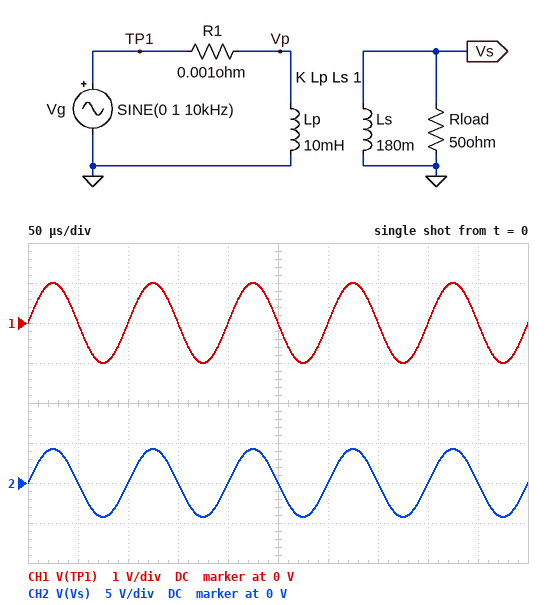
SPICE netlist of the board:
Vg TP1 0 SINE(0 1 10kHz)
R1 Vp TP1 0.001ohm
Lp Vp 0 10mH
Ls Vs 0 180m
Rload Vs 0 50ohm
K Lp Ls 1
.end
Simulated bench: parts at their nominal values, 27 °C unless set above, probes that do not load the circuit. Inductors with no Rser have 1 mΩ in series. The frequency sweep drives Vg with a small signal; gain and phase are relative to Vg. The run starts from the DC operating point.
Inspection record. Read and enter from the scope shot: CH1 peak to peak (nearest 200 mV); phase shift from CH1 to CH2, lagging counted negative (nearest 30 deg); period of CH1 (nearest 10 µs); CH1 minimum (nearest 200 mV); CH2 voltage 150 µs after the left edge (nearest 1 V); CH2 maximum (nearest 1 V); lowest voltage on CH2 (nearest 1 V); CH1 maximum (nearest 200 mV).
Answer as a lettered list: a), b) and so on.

a) 2.0 V
b) 0 deg
c) 100 µs
d) -1.0 V
e) 0 V
f) 4 V
g) -4 V
h) 1.0 V
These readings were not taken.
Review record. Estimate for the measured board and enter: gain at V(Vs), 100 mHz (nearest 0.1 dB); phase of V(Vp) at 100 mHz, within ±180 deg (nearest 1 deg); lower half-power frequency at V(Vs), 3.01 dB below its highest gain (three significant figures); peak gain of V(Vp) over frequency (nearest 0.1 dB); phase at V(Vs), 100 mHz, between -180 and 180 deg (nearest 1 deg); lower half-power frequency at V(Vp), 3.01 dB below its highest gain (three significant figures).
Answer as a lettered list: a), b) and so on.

a) 12.1 dB
b) 9 deg
c) 31.8 mHz
d) 0 dB
e) 18 deg
f) 22.5 mHz
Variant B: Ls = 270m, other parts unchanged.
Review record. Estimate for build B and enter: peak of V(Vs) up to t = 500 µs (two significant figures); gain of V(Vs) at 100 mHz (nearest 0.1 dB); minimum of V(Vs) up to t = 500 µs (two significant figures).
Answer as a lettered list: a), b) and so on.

a) 5.2 V
b) 13.9 dB
c) -5.2 V
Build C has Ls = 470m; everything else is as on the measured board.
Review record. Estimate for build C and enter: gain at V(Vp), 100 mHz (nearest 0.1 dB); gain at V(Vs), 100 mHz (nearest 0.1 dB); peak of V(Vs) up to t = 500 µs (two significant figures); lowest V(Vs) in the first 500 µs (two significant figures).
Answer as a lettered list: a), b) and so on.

a) -0.3 dB
b) 16.3 dB
c) 6.8 V
d) -6.8 V
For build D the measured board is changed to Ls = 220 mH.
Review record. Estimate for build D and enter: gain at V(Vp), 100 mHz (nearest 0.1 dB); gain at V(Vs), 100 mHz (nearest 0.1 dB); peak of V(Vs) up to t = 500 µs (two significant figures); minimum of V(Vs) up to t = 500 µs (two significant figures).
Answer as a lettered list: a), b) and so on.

a) -0.3 dB
b) 13.0 dB
c) 4.7 V
d) -4.7 V
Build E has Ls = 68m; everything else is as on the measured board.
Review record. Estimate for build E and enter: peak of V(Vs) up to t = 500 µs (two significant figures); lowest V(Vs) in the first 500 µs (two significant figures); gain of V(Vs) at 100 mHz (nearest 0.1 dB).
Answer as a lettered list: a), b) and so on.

a) 2.6 V
b) -2.6 V
c) 7.9 dB
